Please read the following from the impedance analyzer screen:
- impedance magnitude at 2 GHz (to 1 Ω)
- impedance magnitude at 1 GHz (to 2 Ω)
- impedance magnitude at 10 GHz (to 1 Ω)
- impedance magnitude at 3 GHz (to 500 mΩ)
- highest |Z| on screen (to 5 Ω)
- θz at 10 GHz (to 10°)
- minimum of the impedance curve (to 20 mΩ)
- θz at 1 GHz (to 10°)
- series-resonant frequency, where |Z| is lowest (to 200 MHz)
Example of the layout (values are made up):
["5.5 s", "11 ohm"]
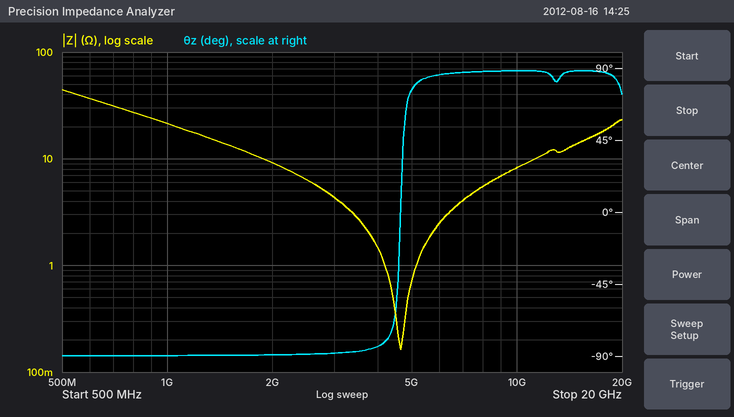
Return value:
["9 Ω", "22 Ω", "8 Ω", "4.5 Ω", "45 Ω", "90°", "160 mΩ", "-90°", "4.6 GHz"]
